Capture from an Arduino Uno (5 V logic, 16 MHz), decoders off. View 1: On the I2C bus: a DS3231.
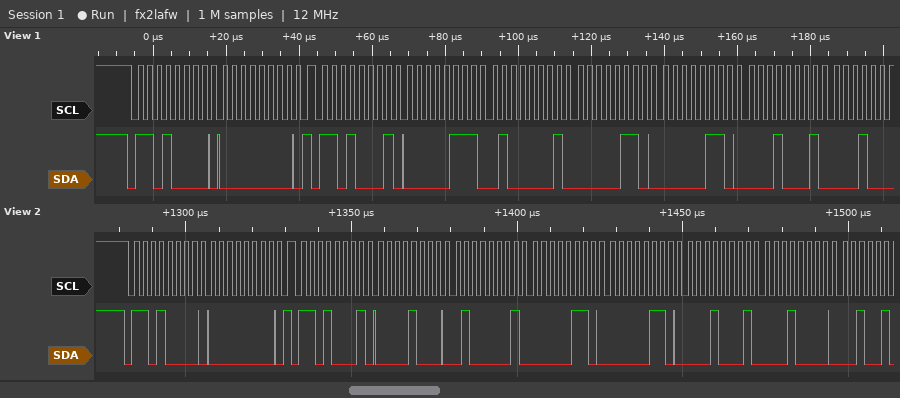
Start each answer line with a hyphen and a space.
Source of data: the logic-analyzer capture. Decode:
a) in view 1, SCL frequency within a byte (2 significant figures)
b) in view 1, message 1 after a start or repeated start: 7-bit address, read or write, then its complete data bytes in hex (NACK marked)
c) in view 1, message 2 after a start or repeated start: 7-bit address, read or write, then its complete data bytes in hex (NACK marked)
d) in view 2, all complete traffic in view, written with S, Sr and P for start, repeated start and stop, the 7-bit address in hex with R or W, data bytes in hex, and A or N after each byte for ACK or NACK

- 400 kHz
- 0x68 write: 00
- 0x68 read: 07 41 06 06 11
- S 68W A 00 A Sr 68R A 08 A 41 A 06 A 06 A 11 A 10 A
